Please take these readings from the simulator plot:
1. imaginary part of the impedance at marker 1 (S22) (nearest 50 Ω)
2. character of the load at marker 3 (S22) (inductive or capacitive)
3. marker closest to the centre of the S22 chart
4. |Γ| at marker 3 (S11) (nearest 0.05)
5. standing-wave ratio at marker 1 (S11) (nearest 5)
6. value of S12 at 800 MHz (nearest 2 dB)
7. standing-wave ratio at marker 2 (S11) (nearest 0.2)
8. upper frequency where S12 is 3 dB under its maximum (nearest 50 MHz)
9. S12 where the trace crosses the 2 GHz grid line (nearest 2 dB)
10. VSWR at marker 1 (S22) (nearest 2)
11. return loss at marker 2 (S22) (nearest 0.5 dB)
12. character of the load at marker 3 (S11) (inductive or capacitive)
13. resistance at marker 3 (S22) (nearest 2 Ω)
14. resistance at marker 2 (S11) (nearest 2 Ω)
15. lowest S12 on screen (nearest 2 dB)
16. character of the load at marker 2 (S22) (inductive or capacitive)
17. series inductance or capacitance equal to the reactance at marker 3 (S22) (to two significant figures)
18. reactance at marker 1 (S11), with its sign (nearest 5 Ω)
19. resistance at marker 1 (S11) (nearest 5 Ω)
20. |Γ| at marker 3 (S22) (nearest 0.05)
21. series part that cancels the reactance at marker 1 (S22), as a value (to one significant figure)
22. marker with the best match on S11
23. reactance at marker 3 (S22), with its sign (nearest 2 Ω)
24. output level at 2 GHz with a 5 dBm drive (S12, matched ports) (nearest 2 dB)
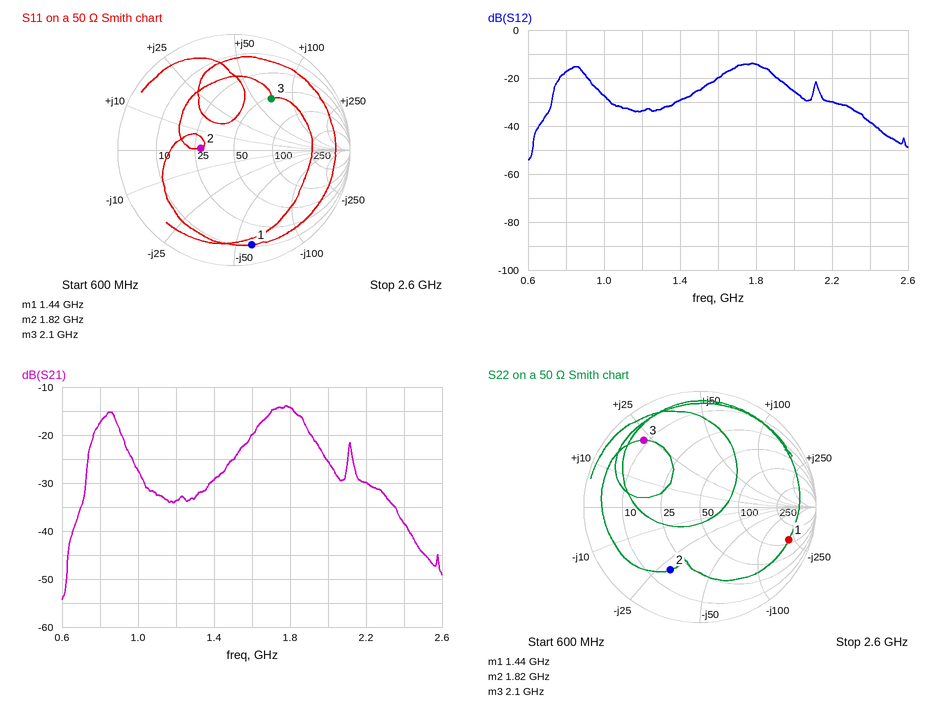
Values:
-200 Ω
inductive
marker 2
0.55
10
-18 dB
1.8
1.85 GHz
-26 dB
10
4.5 dB
inductive
8 Ω
28 Ω
-54 dB
capacitive
1.7 nH
-60 Ω
10 Ω
0.75
20 nH
marker 2
+22 Ω
-20 dBm
